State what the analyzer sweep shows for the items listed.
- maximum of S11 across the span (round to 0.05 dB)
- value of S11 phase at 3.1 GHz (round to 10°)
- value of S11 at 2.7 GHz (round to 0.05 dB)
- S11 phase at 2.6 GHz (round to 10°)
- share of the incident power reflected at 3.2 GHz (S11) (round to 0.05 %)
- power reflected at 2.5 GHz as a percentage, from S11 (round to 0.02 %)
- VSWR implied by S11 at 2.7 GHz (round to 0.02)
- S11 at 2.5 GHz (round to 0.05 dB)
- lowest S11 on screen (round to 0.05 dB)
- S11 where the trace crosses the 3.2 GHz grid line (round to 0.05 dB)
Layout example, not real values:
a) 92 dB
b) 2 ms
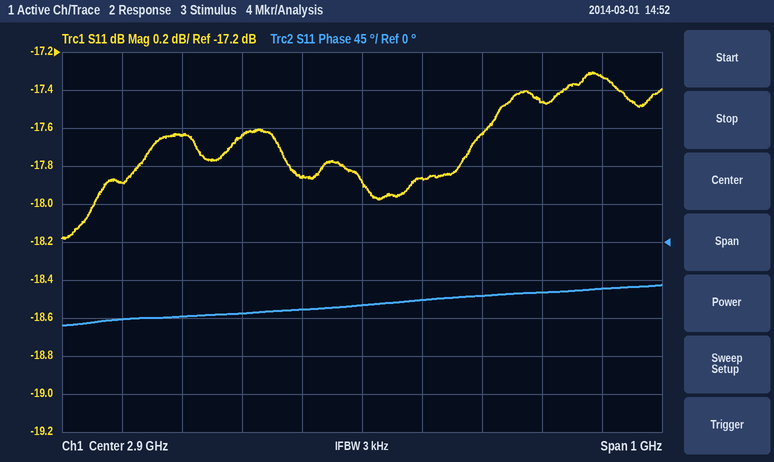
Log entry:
a) -17.30 dB
b) -60°
c) -17.65 dB
d) -90°
e) 1.80 %
f) 1.62 %
g) 1.30
h) -17.90 dB
i) -18.20 dB
j) -17.45 dB
